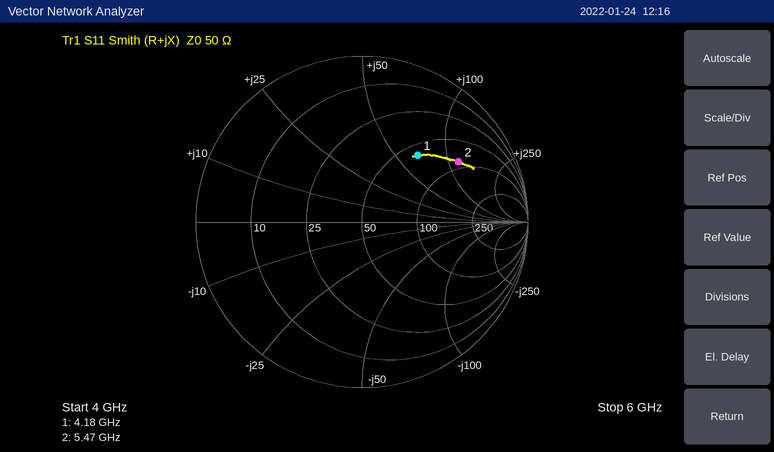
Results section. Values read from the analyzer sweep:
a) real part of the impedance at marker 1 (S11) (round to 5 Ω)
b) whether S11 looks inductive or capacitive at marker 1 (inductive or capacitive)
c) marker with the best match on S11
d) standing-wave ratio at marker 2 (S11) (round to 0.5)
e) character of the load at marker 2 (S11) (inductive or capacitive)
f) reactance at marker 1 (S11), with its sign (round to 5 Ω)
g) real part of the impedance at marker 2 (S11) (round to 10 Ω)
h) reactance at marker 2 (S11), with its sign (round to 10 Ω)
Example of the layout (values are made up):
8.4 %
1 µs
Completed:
60 Ω
inductive
marker 1
5.5
inductive
+65 Ω
90 Ω
+120 Ω
